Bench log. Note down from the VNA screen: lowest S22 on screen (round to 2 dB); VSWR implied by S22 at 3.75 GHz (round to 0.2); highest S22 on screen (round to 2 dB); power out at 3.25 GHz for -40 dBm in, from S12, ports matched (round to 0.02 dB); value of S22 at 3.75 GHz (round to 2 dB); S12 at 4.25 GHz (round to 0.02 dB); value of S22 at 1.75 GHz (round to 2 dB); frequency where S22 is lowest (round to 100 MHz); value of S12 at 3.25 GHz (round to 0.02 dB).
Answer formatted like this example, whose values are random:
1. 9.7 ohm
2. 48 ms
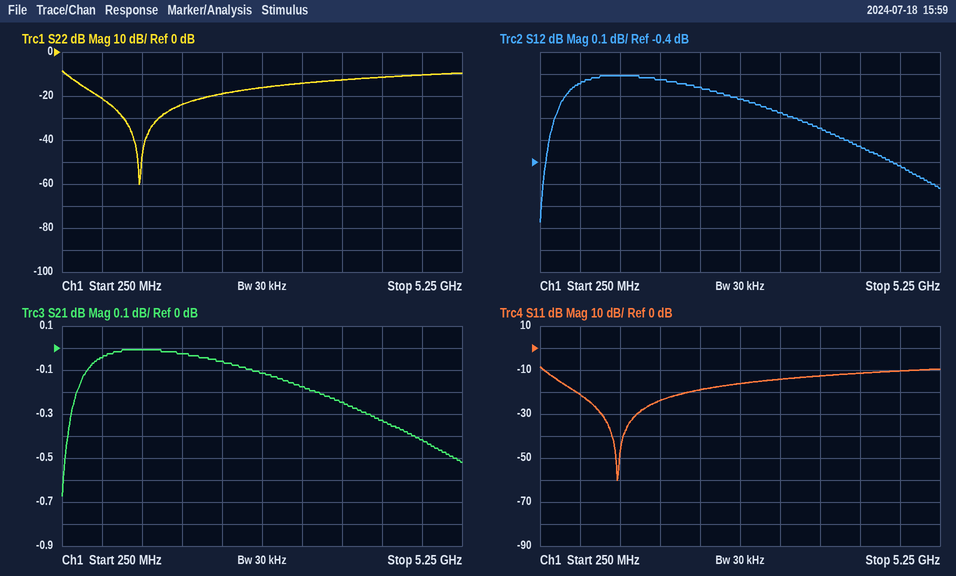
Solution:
1. -60 dB
2. 1.6
3. -8 dB
4. -40.18 dBm
5. -12 dB
6. -0.32 dB
7. -24 dB
8. 1.2 GHz
9. -0.18 dB
